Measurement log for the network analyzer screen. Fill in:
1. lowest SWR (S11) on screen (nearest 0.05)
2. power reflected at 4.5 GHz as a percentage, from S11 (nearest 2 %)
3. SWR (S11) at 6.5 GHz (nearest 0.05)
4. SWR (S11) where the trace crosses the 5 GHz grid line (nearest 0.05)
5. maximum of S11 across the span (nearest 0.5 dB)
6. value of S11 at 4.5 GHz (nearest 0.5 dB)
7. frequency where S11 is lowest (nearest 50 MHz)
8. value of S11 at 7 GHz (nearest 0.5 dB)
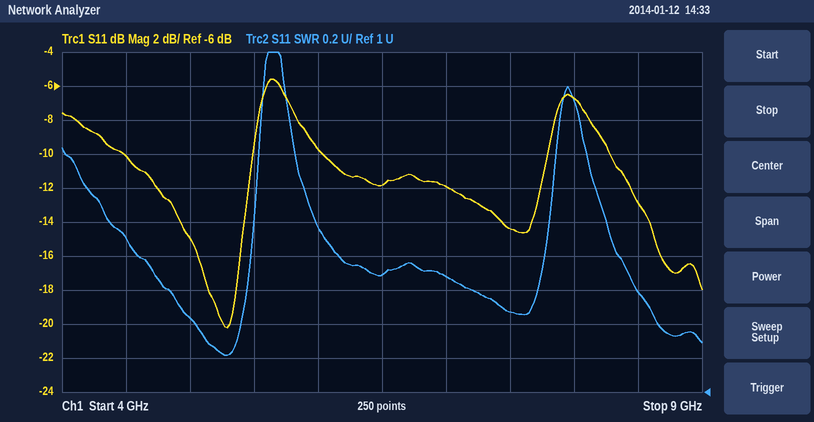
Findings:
1.20
10 %
1.70
1.45
-5.5 dB
-10.0 dB
5.30 GHz
-12.0 dB
